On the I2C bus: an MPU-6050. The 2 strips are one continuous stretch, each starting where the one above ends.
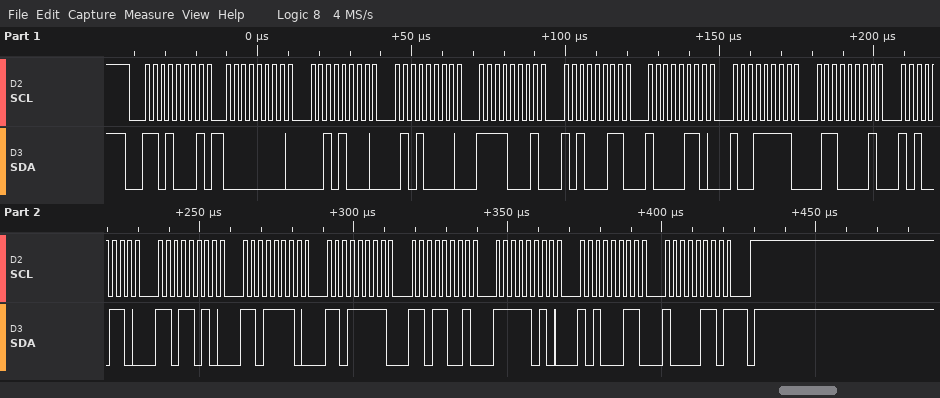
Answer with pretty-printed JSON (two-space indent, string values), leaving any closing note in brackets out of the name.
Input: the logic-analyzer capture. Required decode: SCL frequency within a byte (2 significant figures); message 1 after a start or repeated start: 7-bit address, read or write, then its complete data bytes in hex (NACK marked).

{
  "SCL frequency within a byte": "400 kHz",
  "message 1 after a start or repeated start: 7-bit address, read or write, then its complete data bytes in hex": "0x68 read: 00 28 50 F1 A3 86 9F 61 A6 DA DE DF D9 FA A3 86 NACK"
}
